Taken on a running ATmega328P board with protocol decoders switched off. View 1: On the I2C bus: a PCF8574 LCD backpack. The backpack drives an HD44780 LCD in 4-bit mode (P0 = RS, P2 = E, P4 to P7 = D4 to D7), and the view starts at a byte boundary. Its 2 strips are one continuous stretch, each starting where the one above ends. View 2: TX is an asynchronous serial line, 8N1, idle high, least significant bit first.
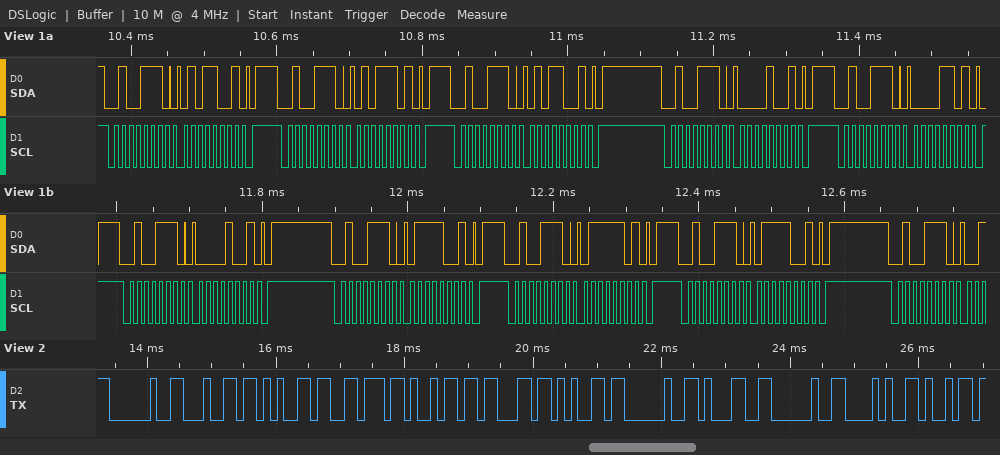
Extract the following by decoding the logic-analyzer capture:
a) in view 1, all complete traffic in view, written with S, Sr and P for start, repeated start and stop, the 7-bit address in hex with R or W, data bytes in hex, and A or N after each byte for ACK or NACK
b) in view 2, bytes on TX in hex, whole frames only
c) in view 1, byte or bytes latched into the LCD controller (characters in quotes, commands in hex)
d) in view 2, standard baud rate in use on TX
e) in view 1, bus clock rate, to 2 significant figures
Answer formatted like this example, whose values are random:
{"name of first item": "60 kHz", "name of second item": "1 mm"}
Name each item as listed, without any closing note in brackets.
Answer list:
{"in view 1, all complete traffic in view, written with S, Sr and P for start, repeated start and stop, the 7-bit address in hex with R or W, data bytes in hex, and A or N after each byte for ACK or NACK": "S 27W A 59 A P S 27W A 5D A P S 27W A 59 A P S 27W A 09 A P S 27W A 0D A P S 27W A 09 A P S 27W A 79 A P S 27W A 7D A P S 27W A 79 A P S 27W A", "in view 2, bytes on TX in hex, whole frames only": "0x20 0x64 0x65 0x76 0x69 0x63 0x65 0x20 0x31 0x20 0x28 0x69", "in view 1, byte or bytes latched into the LCD controller": "'P'", "in view 2, standard baud rate in use on TX": "9600 baud", "in view 1, bus clock rate, to 2 significant figures": "100 kHz"}
